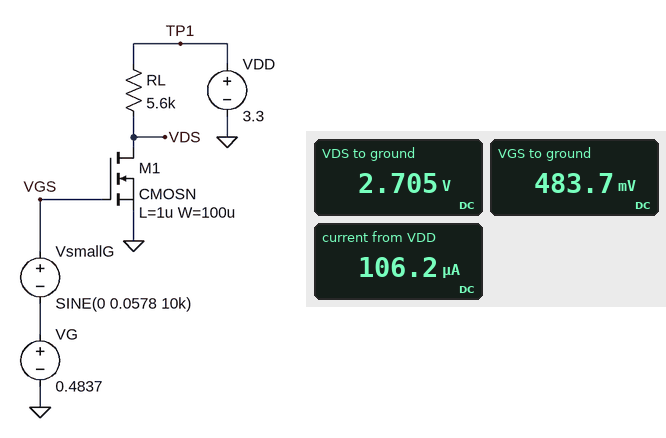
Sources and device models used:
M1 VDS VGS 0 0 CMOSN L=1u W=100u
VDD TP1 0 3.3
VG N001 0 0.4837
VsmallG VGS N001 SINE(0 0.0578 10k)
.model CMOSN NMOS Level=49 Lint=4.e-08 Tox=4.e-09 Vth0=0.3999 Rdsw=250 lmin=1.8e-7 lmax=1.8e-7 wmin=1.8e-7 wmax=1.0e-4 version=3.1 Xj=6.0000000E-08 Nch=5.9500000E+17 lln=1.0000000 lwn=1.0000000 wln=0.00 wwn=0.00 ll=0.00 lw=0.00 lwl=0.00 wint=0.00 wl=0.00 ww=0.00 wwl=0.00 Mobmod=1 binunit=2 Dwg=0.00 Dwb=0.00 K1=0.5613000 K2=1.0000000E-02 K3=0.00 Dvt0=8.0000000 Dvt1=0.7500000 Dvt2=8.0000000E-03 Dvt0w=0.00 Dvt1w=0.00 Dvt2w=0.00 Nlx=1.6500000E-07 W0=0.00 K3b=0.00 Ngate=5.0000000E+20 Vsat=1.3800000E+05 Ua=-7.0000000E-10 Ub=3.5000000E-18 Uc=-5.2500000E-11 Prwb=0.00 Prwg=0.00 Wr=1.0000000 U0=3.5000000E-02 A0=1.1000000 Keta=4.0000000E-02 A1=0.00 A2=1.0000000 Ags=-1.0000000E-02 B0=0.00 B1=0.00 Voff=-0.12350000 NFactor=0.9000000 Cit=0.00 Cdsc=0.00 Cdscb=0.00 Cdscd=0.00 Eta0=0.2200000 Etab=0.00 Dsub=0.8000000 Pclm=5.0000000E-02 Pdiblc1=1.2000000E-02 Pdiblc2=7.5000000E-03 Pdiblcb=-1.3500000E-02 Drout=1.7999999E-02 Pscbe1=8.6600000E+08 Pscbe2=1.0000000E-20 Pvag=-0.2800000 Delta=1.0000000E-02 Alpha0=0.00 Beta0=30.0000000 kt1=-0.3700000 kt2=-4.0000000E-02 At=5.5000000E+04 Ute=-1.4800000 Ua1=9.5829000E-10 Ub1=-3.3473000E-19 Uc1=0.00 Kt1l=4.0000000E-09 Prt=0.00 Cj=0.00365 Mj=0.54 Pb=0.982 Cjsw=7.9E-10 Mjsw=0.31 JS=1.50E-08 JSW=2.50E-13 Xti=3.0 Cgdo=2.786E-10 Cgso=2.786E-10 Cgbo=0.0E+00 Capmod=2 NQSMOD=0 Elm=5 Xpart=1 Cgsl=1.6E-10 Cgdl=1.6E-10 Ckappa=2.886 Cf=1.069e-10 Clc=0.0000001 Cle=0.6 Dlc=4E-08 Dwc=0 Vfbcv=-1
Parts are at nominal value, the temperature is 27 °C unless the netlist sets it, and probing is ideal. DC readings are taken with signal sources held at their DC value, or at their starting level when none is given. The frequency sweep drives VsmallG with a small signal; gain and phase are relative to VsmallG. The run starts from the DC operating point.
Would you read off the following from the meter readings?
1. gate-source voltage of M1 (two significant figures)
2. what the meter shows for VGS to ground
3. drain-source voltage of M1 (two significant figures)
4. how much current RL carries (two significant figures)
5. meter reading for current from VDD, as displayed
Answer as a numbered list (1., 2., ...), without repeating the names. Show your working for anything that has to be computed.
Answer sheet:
1. 483.7 mV = 480 mV
2. 483.7 mV
3. 2.705 V = 2.7 V
4. (3.3 V - 2.705 V) / 5.6 kΩ = 110 µA
5. 106.2 µA
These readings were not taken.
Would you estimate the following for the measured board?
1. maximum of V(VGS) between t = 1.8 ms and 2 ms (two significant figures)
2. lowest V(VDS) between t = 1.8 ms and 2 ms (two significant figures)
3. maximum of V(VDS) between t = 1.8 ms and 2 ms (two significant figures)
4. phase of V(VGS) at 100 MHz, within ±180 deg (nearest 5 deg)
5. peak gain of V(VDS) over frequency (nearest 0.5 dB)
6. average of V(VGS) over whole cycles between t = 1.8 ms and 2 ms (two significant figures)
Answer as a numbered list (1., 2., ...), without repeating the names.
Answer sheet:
1. 540 mV
2. 2.0 V
3. 3.1 V
4. 0 deg
5. 19.5 dB
6. 480 mV
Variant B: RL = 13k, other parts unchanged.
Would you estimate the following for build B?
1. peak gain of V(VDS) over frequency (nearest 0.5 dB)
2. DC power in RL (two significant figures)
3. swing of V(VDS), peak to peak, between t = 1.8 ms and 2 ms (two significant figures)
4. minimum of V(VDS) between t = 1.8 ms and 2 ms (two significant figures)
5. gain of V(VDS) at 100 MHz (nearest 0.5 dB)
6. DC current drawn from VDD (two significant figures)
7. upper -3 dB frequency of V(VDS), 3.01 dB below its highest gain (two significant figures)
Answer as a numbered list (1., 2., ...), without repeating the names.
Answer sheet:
1. 25.5 dB
2. 130 µW
3. 2.1 V
4. 680 mV
5. 23.5 dB
6. 99 µA
7. 130 MHz
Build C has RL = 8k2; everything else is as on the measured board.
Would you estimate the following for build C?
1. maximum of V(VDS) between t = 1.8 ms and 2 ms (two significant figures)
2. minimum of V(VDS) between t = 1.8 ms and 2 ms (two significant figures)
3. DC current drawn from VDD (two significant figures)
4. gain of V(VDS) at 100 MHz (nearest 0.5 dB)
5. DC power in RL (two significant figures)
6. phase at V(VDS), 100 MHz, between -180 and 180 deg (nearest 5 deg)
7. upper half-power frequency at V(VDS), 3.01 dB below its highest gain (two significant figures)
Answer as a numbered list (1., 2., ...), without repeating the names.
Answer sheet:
1. 3.0 V
2. 1.5 V
3. 100 µA
4. 21.5 dB
5. 88 µW
6. 155 deg
7. 210 MHz
